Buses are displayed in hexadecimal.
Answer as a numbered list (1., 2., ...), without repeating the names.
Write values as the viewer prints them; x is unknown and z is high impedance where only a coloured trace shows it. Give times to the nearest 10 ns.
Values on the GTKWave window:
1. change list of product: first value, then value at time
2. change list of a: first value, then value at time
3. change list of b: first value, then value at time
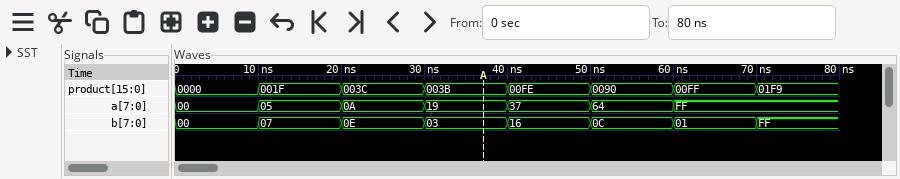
1. 0000, 001F at 10 ns, 003C at 20 ns, 003B at 30 ns, 00FE at 40 ns, 0090 at 50 ns, 00FF at 60 ns, 01F9 at 70 ns
2. 00, 05 at 10 ns, 0A at 20 ns, 19 at 30 ns, 37 at 40 ns, 64 at 50 ns, FF at 60 ns
3. 00, 07 at 10 ns, 0E at 20 ns, 03 at 30 ns, 16 at 40 ns, 0C at 50 ns, 01 at 60 ns, FF at 70 ns
